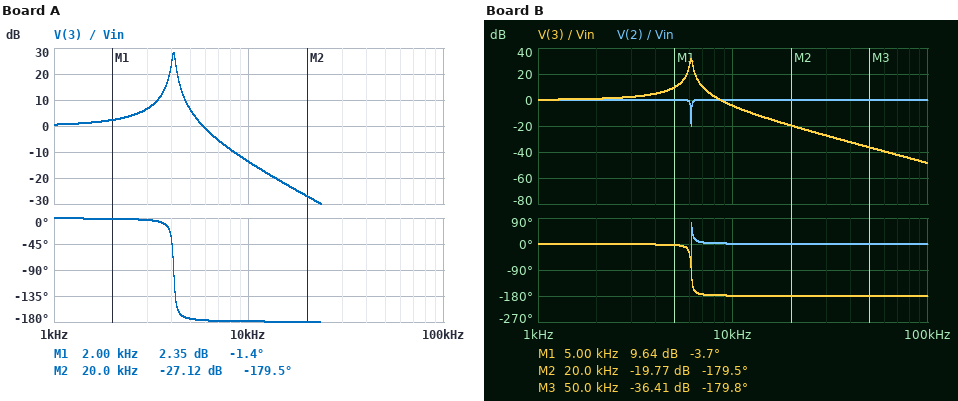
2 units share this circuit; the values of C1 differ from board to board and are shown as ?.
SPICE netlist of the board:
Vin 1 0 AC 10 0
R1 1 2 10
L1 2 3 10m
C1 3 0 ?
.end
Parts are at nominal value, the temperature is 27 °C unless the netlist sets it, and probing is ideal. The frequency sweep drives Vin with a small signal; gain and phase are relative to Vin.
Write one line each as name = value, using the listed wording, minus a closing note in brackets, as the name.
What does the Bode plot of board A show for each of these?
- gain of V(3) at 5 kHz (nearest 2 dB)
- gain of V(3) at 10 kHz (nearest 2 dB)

gain of V(3) at 5 kHz = 6 dB
gain of V(3) at 10 kHz = -14 dB
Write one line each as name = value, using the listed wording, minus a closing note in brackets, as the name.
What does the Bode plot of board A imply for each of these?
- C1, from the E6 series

C1, from the E6 series = 150 nF
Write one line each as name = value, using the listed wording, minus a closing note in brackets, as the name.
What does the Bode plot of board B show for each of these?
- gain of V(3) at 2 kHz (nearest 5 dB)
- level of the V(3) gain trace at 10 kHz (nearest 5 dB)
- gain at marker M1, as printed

gain of V(3) at 2 kHz = 0 dB
level of the V(3) gain trace at 10 kHz = -5 dB
gain at marker M1, as printed = 9.64 dB
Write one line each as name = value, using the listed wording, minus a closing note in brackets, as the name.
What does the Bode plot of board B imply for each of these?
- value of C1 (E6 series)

value of C1 = 68 nF
